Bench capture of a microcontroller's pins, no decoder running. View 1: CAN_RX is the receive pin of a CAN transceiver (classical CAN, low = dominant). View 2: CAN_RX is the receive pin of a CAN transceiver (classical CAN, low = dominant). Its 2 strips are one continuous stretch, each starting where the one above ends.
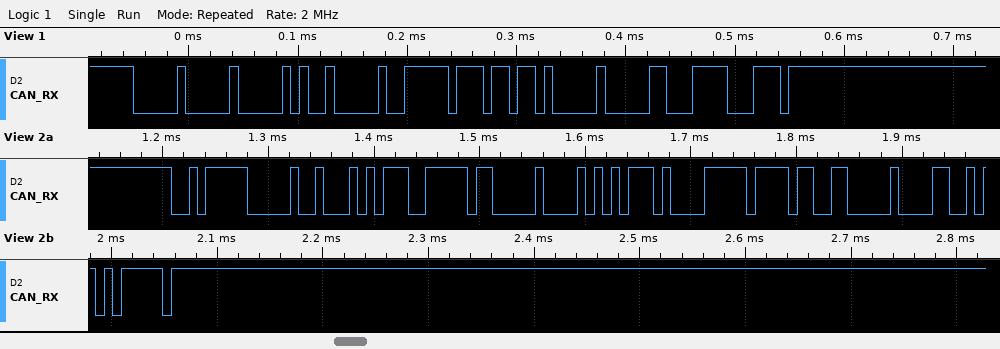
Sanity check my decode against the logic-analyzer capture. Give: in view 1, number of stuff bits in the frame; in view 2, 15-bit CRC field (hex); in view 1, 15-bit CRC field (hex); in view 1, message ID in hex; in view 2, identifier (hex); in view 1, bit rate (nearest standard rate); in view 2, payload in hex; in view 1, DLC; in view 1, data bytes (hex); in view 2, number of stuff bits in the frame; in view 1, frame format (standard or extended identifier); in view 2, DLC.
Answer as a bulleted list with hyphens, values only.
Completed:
- 7
- 0x32AF
- 0x11E3
- 0x000
- 0x2F8
- 125 kbit/s
- AE 7F 00 55 D0 FF B3 00
- 4
- 80 FF 6D 00
- 6
- standard
- 8
